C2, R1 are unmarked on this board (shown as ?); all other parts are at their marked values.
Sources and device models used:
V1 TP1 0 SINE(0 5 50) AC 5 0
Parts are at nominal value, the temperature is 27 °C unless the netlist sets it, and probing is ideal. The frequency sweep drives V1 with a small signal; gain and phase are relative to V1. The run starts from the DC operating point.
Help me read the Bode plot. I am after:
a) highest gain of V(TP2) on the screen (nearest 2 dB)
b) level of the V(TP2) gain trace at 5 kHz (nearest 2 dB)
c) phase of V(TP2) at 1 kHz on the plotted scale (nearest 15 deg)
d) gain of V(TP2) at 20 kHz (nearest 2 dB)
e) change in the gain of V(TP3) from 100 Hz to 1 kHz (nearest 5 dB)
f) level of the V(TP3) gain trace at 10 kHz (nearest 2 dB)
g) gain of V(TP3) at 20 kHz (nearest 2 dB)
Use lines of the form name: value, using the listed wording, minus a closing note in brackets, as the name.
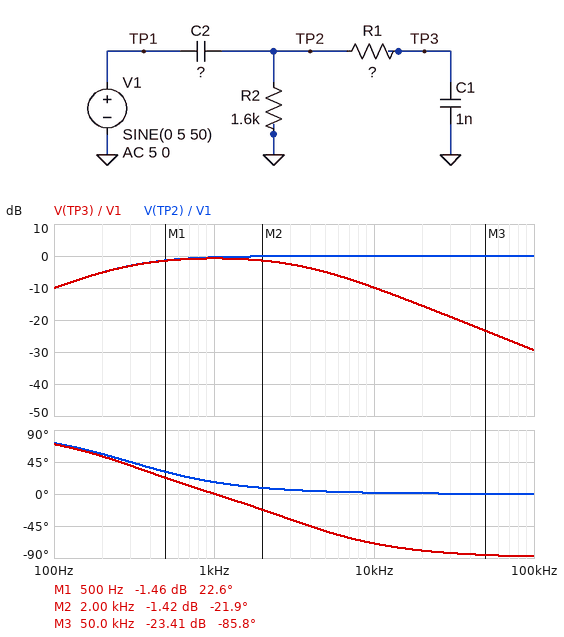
highest gain of V(TP2) on the screen: 0 dB
level of the V(TP2) gain trace at 5 kHz: 0 dB
phase of V(TP2) at 1 kHz on the plotted scale: 15 deg
gain of V(TP2) at 20 kHz: 0 dB
change in the gain of V(TP3) from 100 Hz to 1 kHz: 10 dB
level of the V(TP3) gain trace at 10 kHz: -10 dB
gain of V(TP3) at 20 kHz: -16 dB
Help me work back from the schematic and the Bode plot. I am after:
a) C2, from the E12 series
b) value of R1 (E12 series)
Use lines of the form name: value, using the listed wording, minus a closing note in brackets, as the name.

C2, from the E12 series: 330 nF
value of R1: 47 kΩ
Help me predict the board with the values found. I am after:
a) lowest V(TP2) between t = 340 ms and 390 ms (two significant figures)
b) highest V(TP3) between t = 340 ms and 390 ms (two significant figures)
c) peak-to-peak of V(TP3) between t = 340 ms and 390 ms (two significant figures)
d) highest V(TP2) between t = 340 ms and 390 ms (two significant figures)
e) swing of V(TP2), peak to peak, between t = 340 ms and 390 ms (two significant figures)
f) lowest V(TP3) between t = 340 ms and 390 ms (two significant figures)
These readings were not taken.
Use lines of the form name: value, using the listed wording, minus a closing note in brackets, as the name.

lowest V(TP2) between t = 340 ms and 390 ms: -820 mV
highest V(TP3) between t = 340 ms and 390 ms: 820 mV
peak-to-peak of V(TP3) between t = 340 ms and 390 ms: 1.6 V
highest V(TP2) between t = 340 ms and 390 ms: 820 mV
swing of V(TP2), peak to peak, between t = 340 ms and 390 ms: 1.6 V
lowest V(TP3) between t = 340 ms and 390 ms: -820 mV
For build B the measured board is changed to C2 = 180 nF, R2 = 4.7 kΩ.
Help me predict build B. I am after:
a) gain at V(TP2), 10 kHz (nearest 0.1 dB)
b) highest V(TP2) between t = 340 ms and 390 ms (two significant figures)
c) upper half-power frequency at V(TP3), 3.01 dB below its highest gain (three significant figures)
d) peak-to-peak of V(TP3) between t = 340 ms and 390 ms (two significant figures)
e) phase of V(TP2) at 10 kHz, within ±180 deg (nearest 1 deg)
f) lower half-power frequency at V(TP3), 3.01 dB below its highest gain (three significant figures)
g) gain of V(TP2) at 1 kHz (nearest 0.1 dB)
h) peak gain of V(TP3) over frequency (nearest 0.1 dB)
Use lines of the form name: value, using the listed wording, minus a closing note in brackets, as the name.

gain at V(TP2), 10 kHz: 0 dB
highest V(TP2) between t = 340 ms and 390 ms: 1.3 V
upper half-power frequency at V(TP3), 3.01 dB below its highest gain: 3.76 kHz
peak-to-peak of V(TP3) between t = 340 ms and 390 ms: 2.6 V
phase of V(TP2) at 10 kHz, within ±180 deg: 1 deg
lower half-power frequency at V(TP3), 3.01 dB below its highest gain: 169 Hz
gain of V(TP2) at 1 kHz: -0.2 dB
peak gain of V(TP3) over frequency: -0.5 dB
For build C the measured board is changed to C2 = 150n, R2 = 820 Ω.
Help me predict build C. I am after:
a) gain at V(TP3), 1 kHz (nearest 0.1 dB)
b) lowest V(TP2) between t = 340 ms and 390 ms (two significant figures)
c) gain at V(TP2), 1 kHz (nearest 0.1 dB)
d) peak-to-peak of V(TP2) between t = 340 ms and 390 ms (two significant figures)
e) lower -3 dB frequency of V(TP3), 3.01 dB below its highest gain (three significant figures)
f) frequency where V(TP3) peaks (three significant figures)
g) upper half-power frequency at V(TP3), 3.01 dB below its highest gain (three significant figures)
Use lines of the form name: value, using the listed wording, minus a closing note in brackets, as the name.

gain at V(TP3), 1 kHz: -4.7 dB
lowest V(TP2) between t = 340 ms and 390 ms: -190 mV
gain at V(TP2), 1 kHz: -4.3 dB
peak-to-peak of V(TP2) between t = 340 ms and 390 ms: 390 mV
lower -3 dB frequency of V(TP3), 3.01 dB below its highest gain: 797 Hz
frequency where V(TP3) peaks: 2.09 kHz
upper half-power frequency at V(TP3), 3.01 dB below its highest gain: 5.50 kHz
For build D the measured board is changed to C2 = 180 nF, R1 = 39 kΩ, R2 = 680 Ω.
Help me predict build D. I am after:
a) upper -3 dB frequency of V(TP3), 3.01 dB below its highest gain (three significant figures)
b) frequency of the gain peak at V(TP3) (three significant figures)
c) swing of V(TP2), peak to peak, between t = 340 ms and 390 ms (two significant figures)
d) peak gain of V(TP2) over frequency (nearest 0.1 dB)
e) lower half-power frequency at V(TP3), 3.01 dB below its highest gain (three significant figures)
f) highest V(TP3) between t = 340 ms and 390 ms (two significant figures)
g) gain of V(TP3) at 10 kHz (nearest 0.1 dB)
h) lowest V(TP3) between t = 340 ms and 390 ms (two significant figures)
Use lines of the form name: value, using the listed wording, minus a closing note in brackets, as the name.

upper -3 dB frequency of V(TP3), 3.01 dB below its highest gain: 6.25 kHz
frequency of the gain peak at V(TP3): 2.30 kHz
swing of V(TP2), peak to peak, between t = 340 ms and 390 ms: 380 mV
peak gain of V(TP2) over frequency: 0 dB
lower half-power frequency at V(TP3), 3.01 dB below its highest gain: 849 Hz
highest V(TP3) between t = 340 ms and 390 ms: 190 mV
gain of V(TP3) at 10 kHz: -8.5 dB
lowest V(TP3) between t = 340 ms and 390 ms: -190 mV
